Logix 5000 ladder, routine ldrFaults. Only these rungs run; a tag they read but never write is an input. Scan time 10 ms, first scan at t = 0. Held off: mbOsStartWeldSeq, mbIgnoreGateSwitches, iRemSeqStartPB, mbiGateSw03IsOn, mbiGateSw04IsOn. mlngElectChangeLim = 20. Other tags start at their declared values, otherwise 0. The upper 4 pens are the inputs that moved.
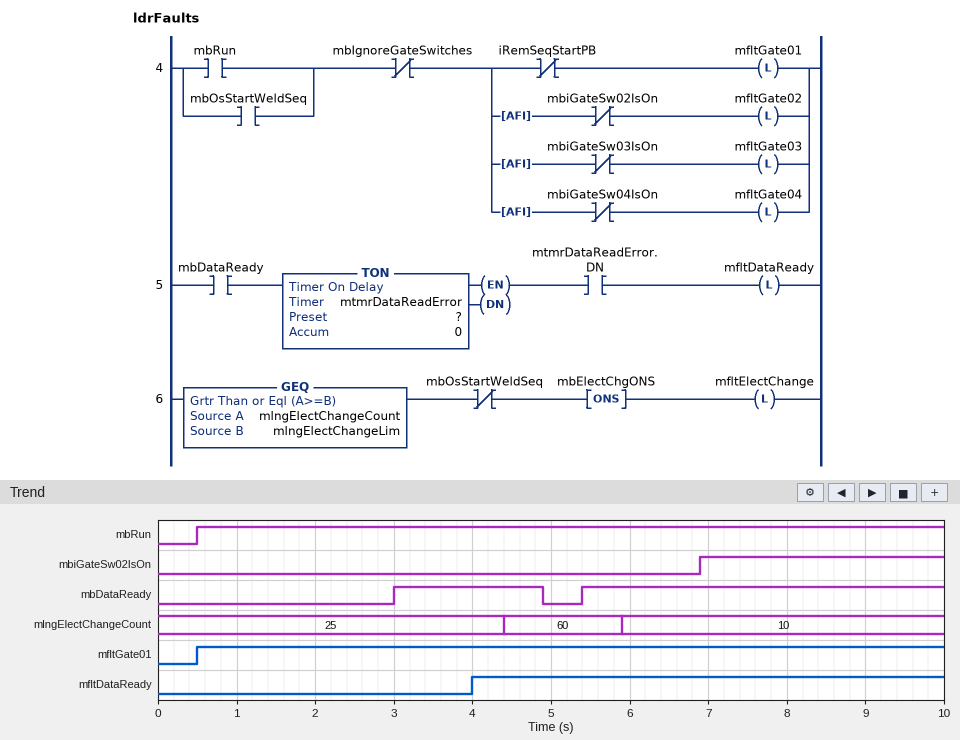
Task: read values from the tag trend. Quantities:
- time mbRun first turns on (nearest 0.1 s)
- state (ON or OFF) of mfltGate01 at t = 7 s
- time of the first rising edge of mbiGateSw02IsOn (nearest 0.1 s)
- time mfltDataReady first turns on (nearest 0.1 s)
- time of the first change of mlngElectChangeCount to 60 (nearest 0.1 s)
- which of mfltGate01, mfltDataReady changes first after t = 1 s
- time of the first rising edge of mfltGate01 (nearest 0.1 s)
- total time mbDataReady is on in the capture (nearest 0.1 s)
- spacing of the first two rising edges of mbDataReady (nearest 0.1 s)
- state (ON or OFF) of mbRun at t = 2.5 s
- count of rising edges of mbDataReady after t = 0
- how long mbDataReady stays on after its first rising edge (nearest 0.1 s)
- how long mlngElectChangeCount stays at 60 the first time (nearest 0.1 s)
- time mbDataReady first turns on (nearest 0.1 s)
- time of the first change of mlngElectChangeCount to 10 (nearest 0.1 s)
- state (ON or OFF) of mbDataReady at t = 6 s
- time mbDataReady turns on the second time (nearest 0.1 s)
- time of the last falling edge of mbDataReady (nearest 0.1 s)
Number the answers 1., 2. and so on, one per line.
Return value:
1. 0.5 s
2. ON
3. 6.9 s
4. 4.0 s
5. 4.4 s
6. mfltDataReady
7. 0.5 s
8. 6.5 s
9. 2.4 s
10. ON
11. 2
12. 1.9 s
13. 1.5 s
14. 3.0 s
15. 5.9 s
16. ON
17. 5.4 s
18. 4.9 s
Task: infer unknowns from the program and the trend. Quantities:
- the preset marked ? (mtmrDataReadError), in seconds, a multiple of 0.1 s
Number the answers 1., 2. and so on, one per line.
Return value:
1. 1.0 s
